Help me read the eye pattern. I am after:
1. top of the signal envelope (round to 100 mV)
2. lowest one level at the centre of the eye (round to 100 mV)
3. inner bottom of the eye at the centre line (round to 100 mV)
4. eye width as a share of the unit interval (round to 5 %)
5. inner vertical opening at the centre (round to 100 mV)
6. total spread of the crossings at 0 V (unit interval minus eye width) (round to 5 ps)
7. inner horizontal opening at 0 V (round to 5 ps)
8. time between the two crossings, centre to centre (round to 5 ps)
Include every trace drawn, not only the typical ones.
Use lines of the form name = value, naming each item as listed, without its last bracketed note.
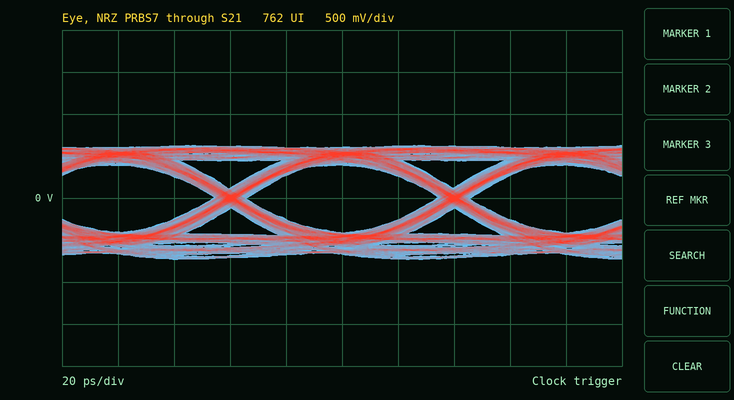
top of the signal envelope = 600 mV
lowest one level at the centre of the eye = 400 mV
inner bottom of the eye at the centre line = -400 mV
eye width as a share of the unit interval = 85 %
inner vertical opening at the centre = 800 mV
total spread of the crossings at 0 V (unit interval minus eye width) = 10 ps
inner horizontal opening at 0 V = 70 ps
time between the two crossings, centre to centre = 80 ps
